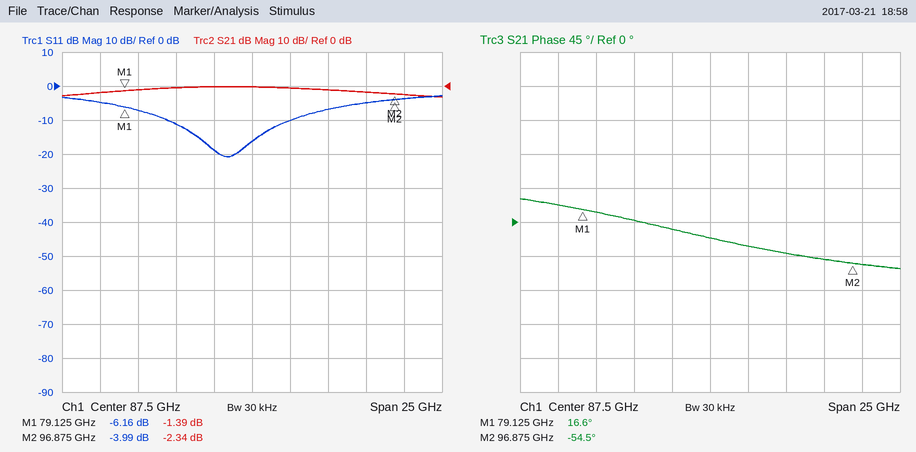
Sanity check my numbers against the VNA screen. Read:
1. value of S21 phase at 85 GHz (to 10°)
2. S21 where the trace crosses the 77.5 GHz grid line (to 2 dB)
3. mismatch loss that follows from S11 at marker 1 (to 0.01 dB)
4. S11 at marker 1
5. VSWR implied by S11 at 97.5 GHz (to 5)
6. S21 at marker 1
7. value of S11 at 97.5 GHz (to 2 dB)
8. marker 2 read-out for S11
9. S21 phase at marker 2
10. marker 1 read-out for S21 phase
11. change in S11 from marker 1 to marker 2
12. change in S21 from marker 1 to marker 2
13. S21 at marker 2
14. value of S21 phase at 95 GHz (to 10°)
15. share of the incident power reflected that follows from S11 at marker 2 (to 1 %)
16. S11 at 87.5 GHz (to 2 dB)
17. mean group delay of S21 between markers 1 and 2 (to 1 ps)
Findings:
-10°
-2 dB
1.20 dB
-6.16 dB
5
-1.39 dB
-4 dB
-3.99 dB
-54.5°
16.6°
2.17 dB
-0.95 dB
-2.34 dB
-50°
40 %
-16 dB
11 ps
